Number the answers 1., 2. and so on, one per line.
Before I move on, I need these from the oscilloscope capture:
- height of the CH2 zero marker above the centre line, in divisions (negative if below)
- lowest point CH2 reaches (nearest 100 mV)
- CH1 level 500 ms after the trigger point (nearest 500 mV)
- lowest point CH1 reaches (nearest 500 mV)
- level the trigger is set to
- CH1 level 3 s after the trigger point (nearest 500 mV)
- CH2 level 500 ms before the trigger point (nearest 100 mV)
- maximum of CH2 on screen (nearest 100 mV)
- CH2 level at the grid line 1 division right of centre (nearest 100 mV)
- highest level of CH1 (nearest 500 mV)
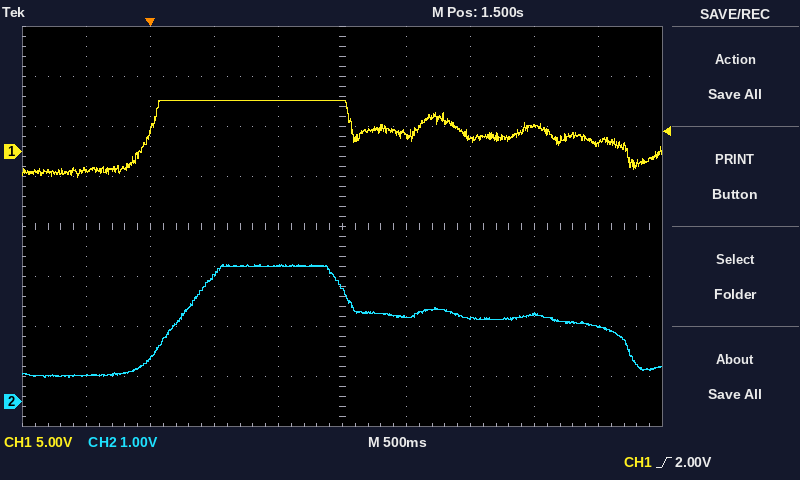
1. -3.5 div
2. 500 mV
3. 5.0 V
4. -2.5 V
5. 2.00 V
6. 2.5 V
7. 500 mV
8. 2.7 V
9. 1.7 V
10. 5.0 V
